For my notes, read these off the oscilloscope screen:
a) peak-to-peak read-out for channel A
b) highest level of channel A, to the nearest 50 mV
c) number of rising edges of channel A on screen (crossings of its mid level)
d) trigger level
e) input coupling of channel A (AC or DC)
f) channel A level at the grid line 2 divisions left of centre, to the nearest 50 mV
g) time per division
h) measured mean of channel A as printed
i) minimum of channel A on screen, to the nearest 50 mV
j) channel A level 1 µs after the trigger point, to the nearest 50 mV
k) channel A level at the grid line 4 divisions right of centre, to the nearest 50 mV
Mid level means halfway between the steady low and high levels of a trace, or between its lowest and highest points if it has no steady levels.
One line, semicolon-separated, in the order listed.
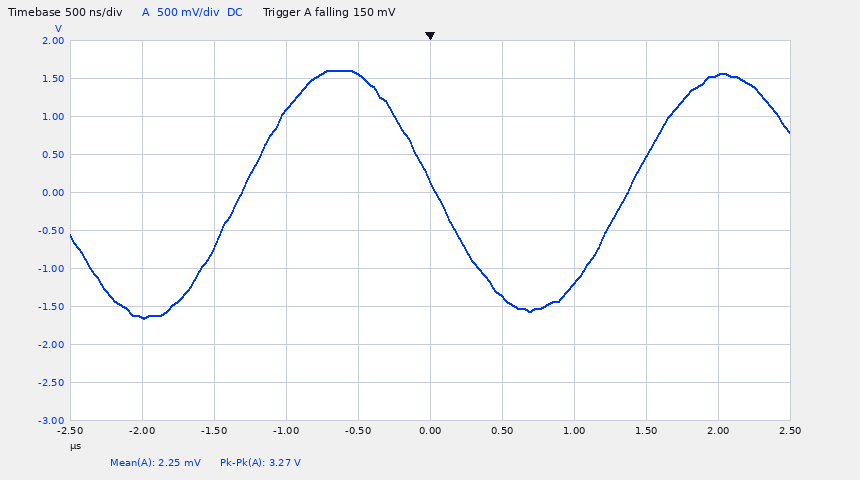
3.27 V; 1.60 V; 2; 150 mV; DC; 1.10 V; 500 ns; 2.25 mV; -1.65 V; -1.20 V; 1.55 V
